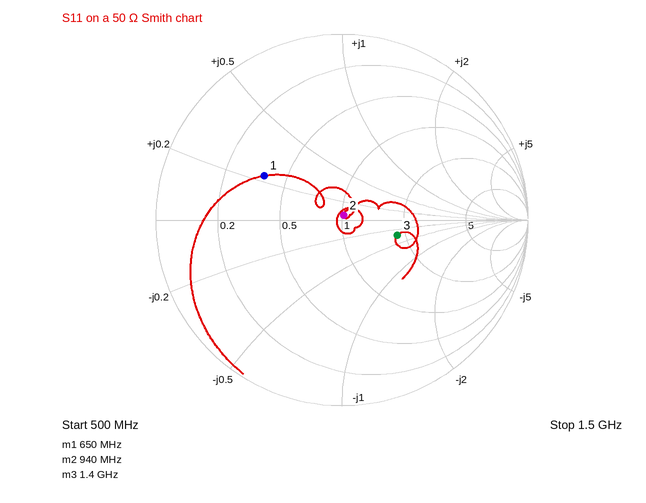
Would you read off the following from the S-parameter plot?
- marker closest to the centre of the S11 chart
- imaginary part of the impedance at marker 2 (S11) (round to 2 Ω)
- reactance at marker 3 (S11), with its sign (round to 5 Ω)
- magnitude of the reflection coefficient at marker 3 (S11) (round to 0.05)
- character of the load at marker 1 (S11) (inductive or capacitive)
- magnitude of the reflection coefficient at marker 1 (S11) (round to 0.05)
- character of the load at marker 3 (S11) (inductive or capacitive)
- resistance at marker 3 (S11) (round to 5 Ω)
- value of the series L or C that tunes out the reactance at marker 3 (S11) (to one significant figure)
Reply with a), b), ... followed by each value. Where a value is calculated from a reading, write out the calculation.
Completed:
a) marker 2
b) +2 Ω
c) -15 Ω
d) 0.30
e) inductive
f) 0.50
g) capacitive
h) 90 Ω
i) L = 15 Ω/(2π × 1.4 GHz) ≈ 2 nH
